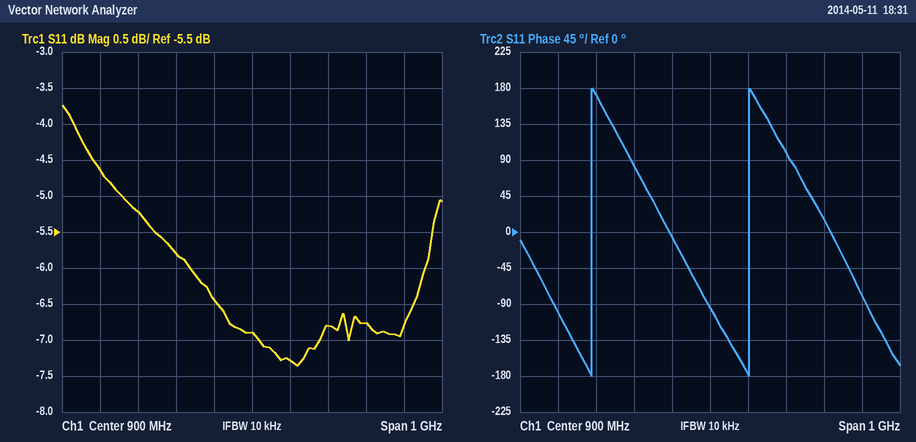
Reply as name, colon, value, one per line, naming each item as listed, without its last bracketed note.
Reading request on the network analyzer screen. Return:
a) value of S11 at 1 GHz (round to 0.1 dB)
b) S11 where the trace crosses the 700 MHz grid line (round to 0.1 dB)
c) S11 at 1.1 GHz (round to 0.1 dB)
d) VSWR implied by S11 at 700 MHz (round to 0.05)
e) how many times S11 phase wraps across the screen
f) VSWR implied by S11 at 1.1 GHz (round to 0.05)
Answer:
value of S11 at 1 GHz: -7.3 dB
S11 where the trace crosses the 700 MHz grid line: -5.8 dB
S11 at 1.1 GHz: -6.8 dB
VSWR implied by S11 at 700 MHz: 3.10
how many times S11 phase wraps across the screen: 2
VSWR implied by S11 at 1.1 GHz: 2.70
